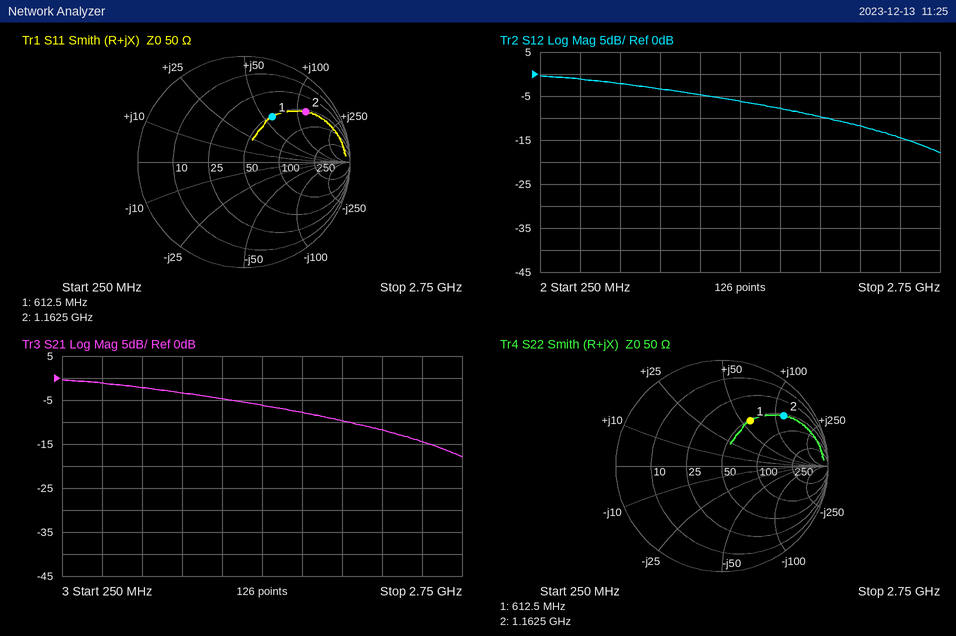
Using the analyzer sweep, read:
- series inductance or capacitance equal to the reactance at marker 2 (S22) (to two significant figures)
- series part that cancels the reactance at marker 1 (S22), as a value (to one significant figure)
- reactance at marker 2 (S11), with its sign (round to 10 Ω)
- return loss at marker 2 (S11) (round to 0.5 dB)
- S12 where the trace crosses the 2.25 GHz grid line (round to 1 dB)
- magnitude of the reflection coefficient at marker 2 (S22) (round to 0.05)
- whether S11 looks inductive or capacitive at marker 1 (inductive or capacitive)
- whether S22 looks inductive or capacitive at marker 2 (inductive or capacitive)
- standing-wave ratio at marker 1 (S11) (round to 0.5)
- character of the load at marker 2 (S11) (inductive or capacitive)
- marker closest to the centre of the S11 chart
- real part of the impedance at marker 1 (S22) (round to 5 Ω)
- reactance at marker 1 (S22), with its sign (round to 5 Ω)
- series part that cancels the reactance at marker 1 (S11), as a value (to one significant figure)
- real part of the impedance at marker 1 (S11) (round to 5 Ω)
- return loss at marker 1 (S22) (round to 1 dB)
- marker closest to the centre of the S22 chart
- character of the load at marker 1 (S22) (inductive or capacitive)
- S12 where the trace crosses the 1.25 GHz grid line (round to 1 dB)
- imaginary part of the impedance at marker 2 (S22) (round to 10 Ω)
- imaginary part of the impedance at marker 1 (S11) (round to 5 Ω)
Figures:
16 nH
4 pF
+120 Ω
2.5 dB
-12 dB
0.75
inductive
inductive
3.0
inductive
marker 1
50 Ω
+60 Ω
4 pF
50 Ω
6 dB
marker 1
inductive
-5 dB
+120 Ω
+60 Ω
